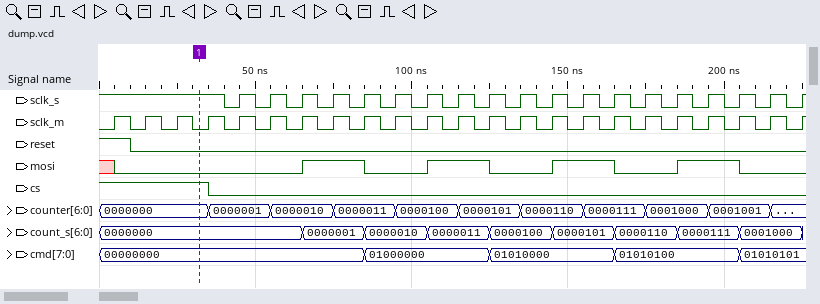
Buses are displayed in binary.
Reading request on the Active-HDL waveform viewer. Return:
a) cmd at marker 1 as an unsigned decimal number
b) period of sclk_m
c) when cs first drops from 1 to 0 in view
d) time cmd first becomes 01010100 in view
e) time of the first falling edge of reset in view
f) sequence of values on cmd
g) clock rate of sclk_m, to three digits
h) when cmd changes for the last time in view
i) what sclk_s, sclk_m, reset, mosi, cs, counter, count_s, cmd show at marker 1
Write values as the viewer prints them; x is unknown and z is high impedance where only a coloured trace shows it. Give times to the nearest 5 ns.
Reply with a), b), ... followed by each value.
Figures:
a) 0
b) 10 ns
c) 35 ns
d) 165 ns
e) 10 ns
f) 00000000, 01000000, 01010000, 01010100, 01010101
g) 100 MHz
h) 205 ns
i) sclk_s=1, sclk_m=0, reset=0, mosi=0, cs=1, counter=0000000, count_s=0000000, cmd=00000000
